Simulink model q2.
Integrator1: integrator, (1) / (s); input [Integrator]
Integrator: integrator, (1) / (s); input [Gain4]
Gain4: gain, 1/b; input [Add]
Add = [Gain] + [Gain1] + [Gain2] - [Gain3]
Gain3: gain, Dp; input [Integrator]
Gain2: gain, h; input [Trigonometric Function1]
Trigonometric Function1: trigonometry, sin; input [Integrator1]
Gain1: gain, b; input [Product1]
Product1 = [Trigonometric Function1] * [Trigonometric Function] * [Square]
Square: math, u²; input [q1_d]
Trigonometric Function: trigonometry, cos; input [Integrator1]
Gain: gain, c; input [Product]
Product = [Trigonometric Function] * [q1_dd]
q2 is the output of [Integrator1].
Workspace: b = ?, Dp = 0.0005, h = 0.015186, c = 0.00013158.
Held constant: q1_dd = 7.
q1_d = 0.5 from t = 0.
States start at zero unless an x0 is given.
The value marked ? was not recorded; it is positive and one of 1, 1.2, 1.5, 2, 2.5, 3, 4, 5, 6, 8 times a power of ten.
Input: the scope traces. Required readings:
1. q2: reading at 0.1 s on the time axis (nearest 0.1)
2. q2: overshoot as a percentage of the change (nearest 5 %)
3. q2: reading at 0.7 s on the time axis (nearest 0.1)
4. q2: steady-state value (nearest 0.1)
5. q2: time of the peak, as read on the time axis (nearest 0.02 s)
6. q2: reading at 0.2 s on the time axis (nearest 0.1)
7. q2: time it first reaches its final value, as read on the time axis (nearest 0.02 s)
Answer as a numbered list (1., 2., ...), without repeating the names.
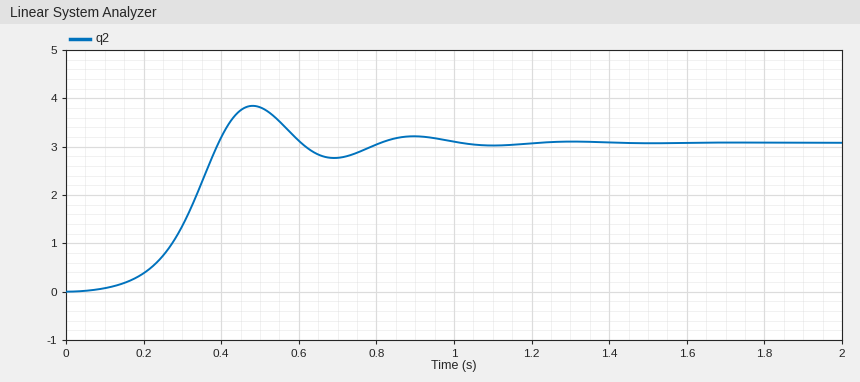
1. 0.1
2. 25 %
3. 2.8
4. 3.1
5. 0.48 s
6. 0.4
7. 0.40 s
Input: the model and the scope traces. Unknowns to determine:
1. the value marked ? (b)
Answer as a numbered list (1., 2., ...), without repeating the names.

1. 6e-05
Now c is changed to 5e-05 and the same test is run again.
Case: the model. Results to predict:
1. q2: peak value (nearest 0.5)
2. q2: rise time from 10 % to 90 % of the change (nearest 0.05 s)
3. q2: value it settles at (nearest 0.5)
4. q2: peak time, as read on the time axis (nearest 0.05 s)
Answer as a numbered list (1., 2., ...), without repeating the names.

1. 4.0
2. 0.20 s
3. 3.0
4. 0.55 s
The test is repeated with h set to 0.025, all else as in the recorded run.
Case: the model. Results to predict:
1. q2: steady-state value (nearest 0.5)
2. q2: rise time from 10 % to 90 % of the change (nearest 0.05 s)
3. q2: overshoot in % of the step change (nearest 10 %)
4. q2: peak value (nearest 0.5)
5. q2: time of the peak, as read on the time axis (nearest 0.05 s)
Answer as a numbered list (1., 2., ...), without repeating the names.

1. 3.0
2. 0.15 s
3. 30 %
4. 4.0
5. 0.40 s
